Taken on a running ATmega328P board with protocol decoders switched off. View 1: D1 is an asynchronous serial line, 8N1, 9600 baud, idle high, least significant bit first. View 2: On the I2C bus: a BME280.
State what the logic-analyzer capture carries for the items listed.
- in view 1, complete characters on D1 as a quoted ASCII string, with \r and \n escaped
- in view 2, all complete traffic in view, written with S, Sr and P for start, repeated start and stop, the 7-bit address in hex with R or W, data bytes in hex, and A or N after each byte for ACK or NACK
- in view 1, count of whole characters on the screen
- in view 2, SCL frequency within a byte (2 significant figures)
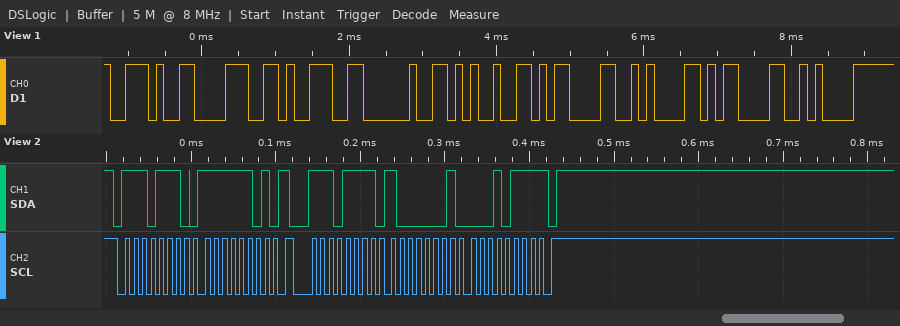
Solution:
".89 %\r\n\r\n"
S 77W A FD A Sr 77R A 81 A 17 N P
9
100 kHz
